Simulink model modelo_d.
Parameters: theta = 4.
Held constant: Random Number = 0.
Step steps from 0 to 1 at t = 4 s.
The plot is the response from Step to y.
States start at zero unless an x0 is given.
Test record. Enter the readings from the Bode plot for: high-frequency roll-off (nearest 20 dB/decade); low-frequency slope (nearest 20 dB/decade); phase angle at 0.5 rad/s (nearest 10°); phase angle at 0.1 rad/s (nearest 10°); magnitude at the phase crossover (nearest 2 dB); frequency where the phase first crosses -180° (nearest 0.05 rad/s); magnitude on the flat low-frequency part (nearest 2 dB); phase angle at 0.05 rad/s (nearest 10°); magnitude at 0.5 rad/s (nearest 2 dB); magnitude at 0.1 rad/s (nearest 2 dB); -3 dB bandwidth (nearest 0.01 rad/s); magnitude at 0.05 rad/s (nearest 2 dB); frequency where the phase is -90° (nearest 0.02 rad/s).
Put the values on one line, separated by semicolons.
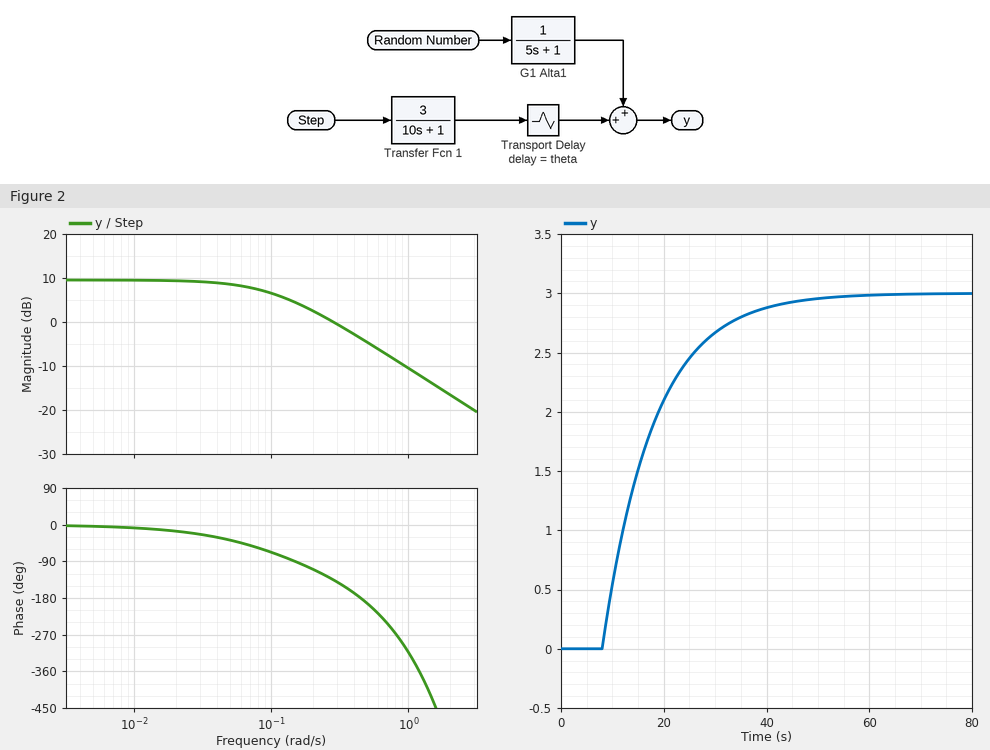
-20 dB/decade; 0 dB/decade; -190°; -70°; -4 dB; 0.45 rad/s; 10 dB; -40°; -4 dB; 6 dB; 0.10 rad/s; 8 dB; 0.14 rad/s
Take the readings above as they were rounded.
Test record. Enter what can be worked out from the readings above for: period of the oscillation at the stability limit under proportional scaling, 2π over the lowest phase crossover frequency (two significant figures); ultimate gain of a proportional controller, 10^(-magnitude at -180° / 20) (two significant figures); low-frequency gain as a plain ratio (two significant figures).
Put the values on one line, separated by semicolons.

14 s; 1.6; 3.2
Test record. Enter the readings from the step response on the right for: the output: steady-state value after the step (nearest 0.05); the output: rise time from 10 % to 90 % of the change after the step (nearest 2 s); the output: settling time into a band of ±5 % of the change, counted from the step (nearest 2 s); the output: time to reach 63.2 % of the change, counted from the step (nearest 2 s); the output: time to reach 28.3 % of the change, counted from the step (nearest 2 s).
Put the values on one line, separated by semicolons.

3.00; 22 s; 34 s; 14 s; 8 s
